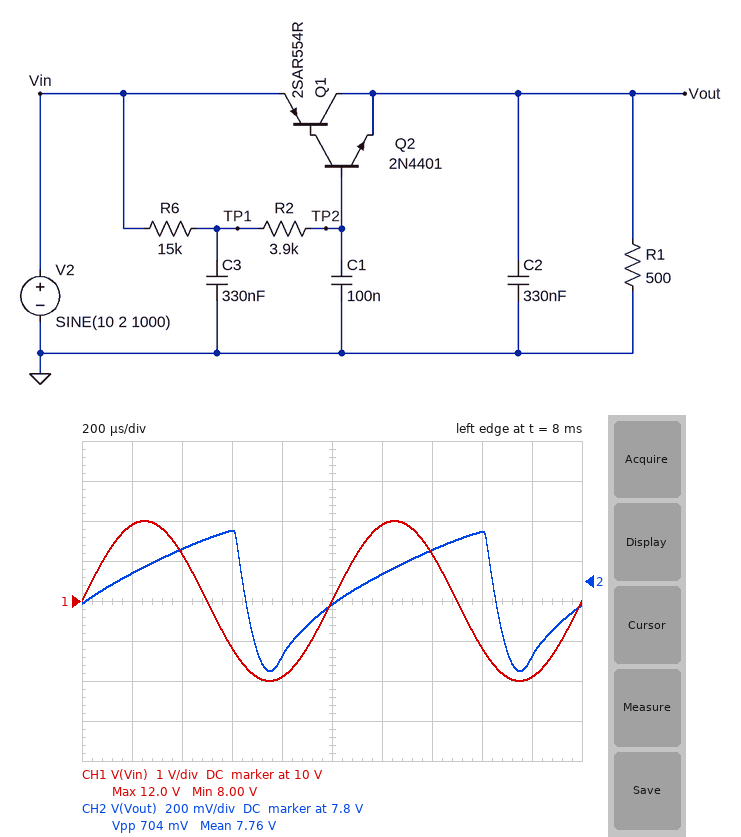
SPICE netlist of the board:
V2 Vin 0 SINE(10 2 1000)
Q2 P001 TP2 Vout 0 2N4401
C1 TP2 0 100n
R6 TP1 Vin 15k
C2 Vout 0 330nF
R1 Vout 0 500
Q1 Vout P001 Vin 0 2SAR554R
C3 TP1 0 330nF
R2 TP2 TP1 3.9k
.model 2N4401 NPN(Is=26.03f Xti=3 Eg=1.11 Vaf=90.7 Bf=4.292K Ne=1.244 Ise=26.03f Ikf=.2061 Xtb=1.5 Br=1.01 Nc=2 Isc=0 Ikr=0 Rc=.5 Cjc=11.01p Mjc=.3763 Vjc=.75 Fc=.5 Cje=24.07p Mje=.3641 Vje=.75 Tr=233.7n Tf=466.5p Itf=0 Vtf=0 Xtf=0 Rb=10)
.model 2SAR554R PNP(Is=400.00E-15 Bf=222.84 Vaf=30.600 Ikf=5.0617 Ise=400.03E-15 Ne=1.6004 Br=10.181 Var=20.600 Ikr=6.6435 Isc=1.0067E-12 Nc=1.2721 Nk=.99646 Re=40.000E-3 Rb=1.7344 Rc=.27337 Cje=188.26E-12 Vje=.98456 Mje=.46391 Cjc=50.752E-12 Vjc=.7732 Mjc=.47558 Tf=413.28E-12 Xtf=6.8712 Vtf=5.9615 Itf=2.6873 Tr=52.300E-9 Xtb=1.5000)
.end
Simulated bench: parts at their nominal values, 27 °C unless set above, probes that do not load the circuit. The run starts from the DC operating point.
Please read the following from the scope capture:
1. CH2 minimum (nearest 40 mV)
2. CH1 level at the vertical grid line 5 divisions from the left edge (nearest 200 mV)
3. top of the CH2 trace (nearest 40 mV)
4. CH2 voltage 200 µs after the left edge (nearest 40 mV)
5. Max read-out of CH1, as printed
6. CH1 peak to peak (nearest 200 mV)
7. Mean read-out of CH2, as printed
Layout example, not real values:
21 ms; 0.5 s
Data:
7.36 V; 10.0 V; 8.04 V; 7.84 V; 12.0 V; 4.0 V; 7.76 V
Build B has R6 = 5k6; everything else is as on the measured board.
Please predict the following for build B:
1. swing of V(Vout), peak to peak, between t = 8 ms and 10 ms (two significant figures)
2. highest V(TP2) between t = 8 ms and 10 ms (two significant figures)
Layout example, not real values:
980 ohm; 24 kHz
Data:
1.1 V; 9.0 V
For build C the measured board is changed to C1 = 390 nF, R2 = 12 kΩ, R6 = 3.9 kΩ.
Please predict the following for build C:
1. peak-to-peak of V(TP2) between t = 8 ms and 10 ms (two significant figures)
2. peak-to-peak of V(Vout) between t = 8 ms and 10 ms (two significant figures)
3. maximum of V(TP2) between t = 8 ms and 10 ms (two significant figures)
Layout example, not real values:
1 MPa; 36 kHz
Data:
260 mV; 320 mV; 8.2 V
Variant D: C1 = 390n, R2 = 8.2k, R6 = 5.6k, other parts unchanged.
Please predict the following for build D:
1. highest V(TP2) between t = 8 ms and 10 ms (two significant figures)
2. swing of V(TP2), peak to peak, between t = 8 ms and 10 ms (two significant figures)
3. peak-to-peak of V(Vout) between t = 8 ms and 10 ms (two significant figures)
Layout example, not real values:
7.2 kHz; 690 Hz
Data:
8.3 V; 300 mV; 360 mV
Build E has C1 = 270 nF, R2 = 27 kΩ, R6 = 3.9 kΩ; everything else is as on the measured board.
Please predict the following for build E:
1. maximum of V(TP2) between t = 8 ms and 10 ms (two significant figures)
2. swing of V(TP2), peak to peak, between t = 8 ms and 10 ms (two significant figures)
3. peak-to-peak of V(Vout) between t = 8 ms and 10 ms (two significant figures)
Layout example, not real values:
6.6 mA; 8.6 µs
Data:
8.2 V; 200 mV; 250 mV
